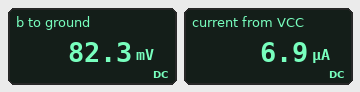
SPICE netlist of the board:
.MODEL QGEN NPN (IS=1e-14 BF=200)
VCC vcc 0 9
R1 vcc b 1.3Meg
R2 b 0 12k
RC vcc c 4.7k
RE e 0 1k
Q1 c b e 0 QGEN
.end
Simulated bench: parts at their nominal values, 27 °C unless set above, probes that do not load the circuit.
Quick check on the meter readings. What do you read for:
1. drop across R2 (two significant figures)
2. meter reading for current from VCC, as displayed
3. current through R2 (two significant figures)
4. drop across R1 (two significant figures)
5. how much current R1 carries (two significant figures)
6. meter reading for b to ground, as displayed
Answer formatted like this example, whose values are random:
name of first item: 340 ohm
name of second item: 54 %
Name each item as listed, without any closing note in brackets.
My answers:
drop across R2: 82 mV
meter reading for current from VCC, as displayed: 6.9 µA
current through R2: 6.9 µA
drop across R1: 8.9 V
how much current R1 carries: 6.9 µA
meter reading for b to ground, as displayed: 82.3 mV
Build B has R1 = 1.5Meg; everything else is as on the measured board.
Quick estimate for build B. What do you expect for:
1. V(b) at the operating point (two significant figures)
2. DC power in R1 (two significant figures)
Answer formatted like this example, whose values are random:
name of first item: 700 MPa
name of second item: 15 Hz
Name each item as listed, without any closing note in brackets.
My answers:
V(b) at the operating point: 71 mV
DC power in R1: 53 µW
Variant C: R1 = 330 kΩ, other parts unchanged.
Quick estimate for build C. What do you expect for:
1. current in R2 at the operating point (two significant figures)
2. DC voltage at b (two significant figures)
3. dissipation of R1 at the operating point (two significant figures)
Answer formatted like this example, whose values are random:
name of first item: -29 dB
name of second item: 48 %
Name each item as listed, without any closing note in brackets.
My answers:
current in R2 at the operating point: 26 µA
DC voltage at b: 320 mV
dissipation of R1 at the operating point: 230 µW
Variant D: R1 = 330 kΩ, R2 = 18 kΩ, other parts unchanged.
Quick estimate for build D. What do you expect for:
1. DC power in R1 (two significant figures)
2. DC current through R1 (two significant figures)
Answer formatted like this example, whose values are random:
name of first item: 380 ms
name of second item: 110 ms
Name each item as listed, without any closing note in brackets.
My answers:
DC power in R1: 220 µW
DC current through R1: 26 µA
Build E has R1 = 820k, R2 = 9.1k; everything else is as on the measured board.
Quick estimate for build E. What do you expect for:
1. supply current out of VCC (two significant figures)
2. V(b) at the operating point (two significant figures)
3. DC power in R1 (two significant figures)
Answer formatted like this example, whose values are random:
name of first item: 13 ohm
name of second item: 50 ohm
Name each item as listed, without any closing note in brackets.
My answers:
supply current out of VCC: 11 µA
V(b) at the operating point: 99 mV
DC power in R1: 97 µW
